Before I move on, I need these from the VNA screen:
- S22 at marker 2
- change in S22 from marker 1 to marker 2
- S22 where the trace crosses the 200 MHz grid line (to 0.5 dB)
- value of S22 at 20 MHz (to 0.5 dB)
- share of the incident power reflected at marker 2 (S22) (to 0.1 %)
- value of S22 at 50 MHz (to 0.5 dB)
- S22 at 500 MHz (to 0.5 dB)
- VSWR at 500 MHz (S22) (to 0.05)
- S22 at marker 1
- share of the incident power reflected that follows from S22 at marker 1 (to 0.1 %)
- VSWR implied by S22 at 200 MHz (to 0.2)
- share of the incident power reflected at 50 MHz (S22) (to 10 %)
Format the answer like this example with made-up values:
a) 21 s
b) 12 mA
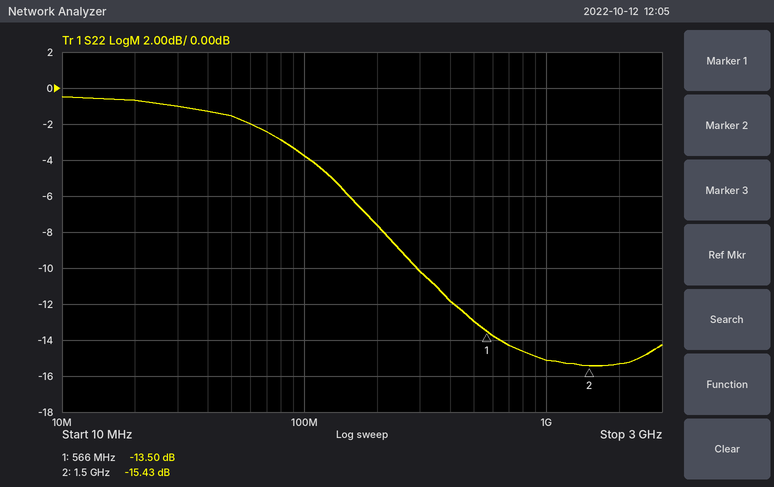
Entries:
a) -15.43 dB
b) -1.93 dB
c) -7.5 dB
d) -0.5 dB
e) 2.9 %
f) -1.5 dB
g) -13.0 dB
h) 1.60
i) -13.50 dB
j) 4.5 %
k) 2.4
l) 70 %
